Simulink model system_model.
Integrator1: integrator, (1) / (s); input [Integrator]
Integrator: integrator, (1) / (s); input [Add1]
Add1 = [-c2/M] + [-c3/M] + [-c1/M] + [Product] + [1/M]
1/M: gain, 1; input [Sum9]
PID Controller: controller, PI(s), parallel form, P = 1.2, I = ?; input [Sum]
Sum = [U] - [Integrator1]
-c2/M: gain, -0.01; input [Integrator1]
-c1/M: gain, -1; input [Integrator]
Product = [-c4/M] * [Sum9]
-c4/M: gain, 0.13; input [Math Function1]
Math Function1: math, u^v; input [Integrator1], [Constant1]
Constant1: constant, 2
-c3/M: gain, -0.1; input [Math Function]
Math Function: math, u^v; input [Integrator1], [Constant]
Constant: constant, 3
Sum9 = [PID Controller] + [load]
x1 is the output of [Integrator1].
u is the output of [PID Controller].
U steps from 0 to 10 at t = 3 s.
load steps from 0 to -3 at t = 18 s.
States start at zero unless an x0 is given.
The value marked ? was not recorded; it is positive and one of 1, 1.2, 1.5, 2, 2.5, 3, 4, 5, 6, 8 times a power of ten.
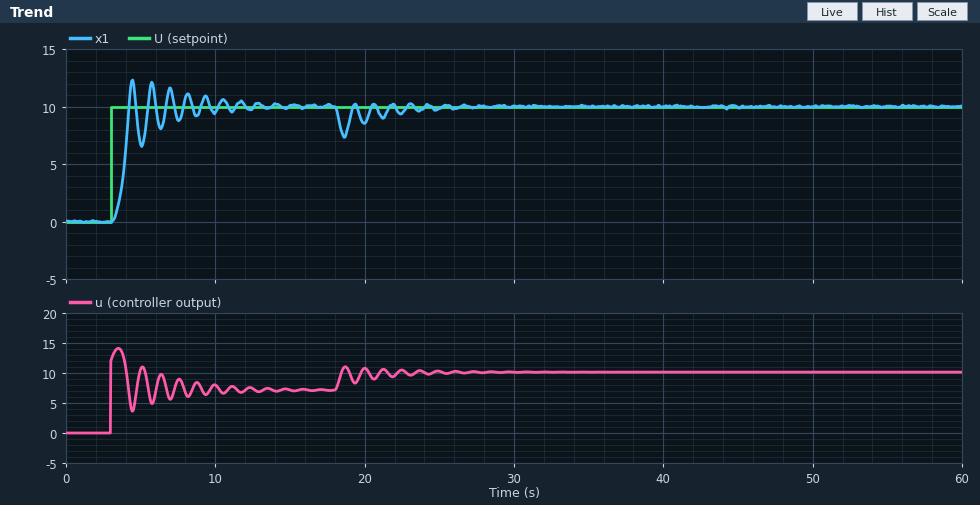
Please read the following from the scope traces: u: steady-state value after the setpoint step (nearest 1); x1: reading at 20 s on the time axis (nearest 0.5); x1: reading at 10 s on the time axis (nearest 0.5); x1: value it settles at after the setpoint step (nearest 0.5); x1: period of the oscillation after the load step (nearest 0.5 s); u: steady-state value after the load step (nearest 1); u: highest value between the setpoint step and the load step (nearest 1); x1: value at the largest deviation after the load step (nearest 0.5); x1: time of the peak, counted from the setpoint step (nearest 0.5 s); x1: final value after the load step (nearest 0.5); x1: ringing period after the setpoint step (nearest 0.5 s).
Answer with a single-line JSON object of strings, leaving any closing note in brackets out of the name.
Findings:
{"u: steady-state value after the setpoint step": "7", "x1: reading at 20 s on the time axis": "8.5", "x1: reading at 10 s on the time axis": "9.5", "x1: value it settles at after the setpoint step": "10.0", "x1: period of the oscillation after the load step": "1.5 s", "u: steady-state value after the load step": "10", "u: highest value between the setpoint step and the load step": "14", "x1: value at the largest deviation after the load step": "7.5", "x1: time of the peak, counted from the setpoint step": "1.5 s", "x1: final value after the load step": "10.0", "x1: ringing period after the setpoint step": "1.5 s"}
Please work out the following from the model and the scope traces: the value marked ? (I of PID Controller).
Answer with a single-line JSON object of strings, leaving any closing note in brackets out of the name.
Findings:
{"the value marked ?": "0.8"}
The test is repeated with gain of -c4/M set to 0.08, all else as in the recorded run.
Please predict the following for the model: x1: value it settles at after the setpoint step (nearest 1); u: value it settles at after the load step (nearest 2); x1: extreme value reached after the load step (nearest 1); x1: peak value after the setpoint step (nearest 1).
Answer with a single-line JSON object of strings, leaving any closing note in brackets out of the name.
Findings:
{"x1: value it settles at after the setpoint step": "10", "u: value it settles at after the load step": "14", "x1: extreme value reached after the load step": "8", "x1: peak value after the setpoint step": "11"}
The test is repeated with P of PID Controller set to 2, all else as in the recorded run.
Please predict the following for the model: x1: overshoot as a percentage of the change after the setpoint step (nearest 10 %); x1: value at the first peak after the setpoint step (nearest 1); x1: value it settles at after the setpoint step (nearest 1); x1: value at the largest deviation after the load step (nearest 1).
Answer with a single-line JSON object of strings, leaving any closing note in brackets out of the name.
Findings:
{"x1: overshoot as a percentage of the change after the setpoint step": "20 %", "x1: value at the first peak after the setpoint step": "12", "x1: value it settles at after the setpoint step": "10", "x1: value at the largest deviation after the load step": "8"}
